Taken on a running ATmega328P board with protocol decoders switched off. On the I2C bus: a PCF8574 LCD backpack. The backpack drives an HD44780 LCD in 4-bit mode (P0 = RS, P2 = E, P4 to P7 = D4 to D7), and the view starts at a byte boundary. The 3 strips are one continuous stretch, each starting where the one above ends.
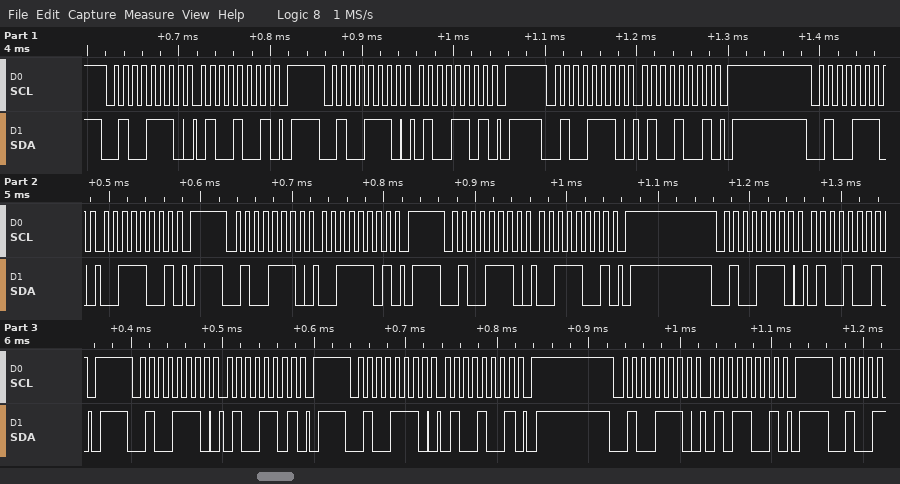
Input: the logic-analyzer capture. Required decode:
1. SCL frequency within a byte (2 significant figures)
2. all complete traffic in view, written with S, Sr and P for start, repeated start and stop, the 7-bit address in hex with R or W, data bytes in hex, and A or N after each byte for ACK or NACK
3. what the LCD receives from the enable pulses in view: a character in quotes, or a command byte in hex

100 kHz
S 27W A 49 A P S 27W A 4D A P S 27W A 49 A P S 27W A 39 A P S 27W A 3D A P S 27W A 39 A P S 27W A 49 A P S 27W A 4D A P S 27W A 49 A P S 27W A 59 A P
'C'
